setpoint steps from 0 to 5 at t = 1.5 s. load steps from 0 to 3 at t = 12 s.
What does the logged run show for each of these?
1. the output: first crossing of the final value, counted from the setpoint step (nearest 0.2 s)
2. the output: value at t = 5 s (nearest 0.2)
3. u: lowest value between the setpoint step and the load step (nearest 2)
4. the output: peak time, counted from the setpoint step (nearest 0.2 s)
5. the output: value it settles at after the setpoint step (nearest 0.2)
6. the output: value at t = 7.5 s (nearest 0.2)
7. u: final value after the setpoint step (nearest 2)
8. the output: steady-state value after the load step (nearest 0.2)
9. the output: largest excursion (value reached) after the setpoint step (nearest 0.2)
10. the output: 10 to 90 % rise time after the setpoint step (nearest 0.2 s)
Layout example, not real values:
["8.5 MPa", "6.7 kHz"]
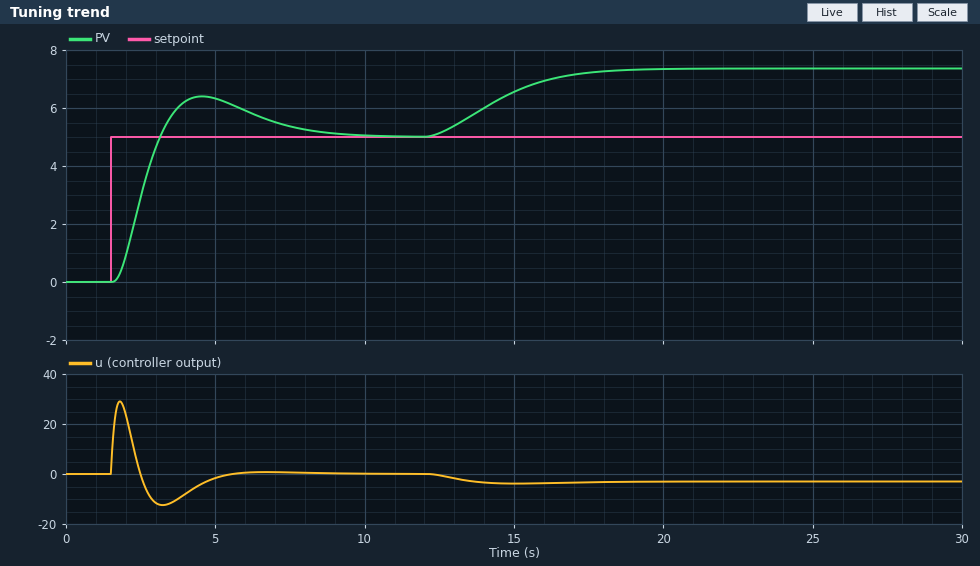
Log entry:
["1.6 s", "6.4", "-12", "3.0 s", "5.0", "5.4", "0", "7.4", "6.4", "1.0 s"]
